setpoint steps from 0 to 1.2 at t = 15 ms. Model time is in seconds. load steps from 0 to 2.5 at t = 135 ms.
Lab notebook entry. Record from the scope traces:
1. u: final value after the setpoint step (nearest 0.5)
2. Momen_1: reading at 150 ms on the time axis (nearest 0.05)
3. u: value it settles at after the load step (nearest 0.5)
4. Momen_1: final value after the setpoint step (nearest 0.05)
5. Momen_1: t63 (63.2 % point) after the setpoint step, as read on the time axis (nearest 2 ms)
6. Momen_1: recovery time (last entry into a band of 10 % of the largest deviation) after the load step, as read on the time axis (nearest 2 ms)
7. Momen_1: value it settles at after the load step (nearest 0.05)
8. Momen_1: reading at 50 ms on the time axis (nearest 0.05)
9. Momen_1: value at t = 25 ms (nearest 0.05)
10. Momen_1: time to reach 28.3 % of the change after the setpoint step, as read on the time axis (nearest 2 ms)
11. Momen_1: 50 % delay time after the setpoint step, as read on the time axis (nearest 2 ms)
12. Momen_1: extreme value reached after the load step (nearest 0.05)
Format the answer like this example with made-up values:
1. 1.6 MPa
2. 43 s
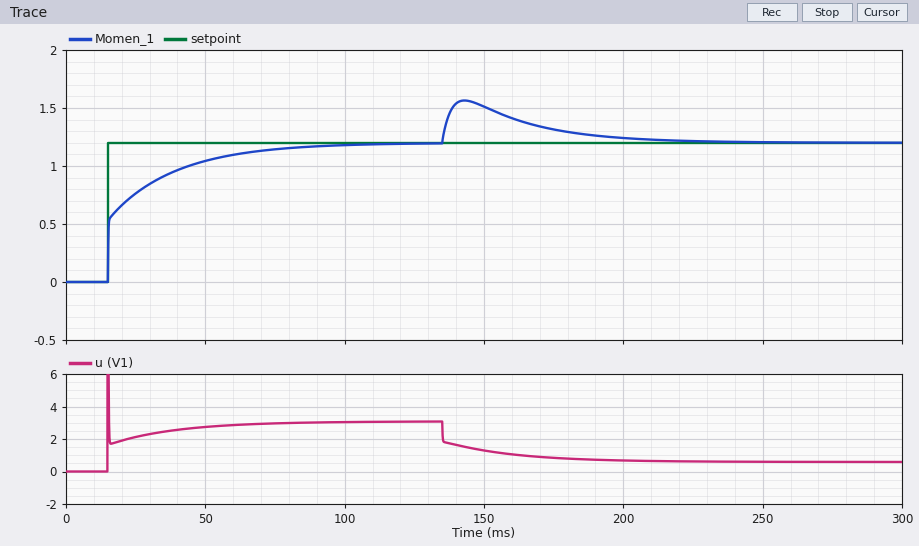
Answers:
1. 3.0
2. 1.50
3. 0.5
4. 1.20
5. 24 ms
6. 202 ms
7. 1.20
8. 1.05
9. 0.75
10. 16 ms
11. 18 ms
12. 1.55
